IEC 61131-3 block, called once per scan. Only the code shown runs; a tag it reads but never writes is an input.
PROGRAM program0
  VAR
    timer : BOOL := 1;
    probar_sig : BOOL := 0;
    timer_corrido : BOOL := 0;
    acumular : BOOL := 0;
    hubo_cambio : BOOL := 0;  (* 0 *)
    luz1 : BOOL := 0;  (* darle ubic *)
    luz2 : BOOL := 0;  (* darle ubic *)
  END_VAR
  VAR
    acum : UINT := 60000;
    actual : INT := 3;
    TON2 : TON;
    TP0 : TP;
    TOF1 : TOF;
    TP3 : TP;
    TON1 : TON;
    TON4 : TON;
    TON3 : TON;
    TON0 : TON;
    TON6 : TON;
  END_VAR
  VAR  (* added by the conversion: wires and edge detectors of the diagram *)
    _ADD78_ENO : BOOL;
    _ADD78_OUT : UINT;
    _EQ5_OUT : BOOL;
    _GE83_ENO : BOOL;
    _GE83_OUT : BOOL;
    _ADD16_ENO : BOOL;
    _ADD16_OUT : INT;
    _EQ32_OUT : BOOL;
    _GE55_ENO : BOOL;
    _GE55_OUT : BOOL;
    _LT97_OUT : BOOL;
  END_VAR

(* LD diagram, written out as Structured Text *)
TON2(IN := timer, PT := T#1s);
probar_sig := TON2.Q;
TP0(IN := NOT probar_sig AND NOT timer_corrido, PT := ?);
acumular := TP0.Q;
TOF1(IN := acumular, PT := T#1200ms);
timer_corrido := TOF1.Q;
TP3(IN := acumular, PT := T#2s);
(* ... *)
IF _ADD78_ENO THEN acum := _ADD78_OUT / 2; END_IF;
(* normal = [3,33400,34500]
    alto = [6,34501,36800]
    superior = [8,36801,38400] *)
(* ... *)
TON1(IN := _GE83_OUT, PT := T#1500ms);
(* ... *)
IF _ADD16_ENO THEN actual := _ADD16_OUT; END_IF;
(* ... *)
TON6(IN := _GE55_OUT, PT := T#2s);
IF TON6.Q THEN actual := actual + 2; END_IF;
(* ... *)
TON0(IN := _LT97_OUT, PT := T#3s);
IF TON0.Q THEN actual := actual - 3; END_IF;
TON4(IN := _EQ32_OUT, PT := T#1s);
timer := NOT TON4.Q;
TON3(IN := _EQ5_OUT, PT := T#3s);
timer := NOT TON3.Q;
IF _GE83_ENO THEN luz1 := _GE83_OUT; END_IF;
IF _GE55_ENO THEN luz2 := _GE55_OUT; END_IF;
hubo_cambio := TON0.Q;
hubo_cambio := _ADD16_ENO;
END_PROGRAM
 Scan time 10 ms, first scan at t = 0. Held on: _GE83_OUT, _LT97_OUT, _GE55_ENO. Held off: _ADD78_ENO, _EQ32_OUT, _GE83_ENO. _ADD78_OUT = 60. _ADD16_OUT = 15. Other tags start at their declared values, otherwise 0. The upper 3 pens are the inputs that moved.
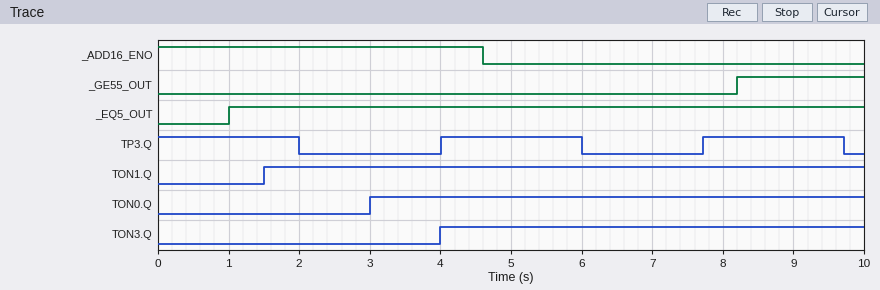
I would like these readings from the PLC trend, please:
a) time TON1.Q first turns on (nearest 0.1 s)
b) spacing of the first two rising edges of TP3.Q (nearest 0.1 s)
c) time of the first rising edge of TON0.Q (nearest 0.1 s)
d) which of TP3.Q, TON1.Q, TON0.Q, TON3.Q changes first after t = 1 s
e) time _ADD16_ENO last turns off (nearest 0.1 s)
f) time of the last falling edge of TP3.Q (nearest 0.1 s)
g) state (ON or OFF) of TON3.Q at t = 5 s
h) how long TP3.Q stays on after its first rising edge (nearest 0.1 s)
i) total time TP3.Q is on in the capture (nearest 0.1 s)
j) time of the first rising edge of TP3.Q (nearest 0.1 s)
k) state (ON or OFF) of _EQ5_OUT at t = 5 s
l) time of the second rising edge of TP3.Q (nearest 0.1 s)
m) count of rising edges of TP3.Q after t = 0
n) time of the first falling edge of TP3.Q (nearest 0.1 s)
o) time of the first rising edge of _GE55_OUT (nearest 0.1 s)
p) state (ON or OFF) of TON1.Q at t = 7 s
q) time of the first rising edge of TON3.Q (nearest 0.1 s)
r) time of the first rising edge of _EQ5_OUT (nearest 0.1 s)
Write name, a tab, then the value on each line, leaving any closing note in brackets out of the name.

time TON1.Q first turns on	1.5 s
spacing of the first two rising edges of TP3.Q	3.7 s
time of the first rising edge of TON0.Q	3.0 s
which of TP3.Q, TON1.Q, TON0.Q, TON3.Q changes first after t = 1 s	TON1.Q
time _ADD16_ENO last turns off	4.6 s
time of the last falling edge of TP3.Q	9.7 s
state (ON or OFF) of TON3.Q at t = 5 s	ON
how long TP3.Q stays on after its first rising edge	2.0 s
total time TP3.Q is on in the capture	6.0 s
time of the first rising edge of TP3.Q	4.0 s
state (ON or OFF) of _EQ5_OUT at t = 5 s	ON
time of the second rising edge of TP3.Q	7.7 s
count of rising edges of TP3.Q after t = 0	2
time of the first falling edge of TP3.Q	2.0 s
time of the first rising edge of _GE55_OUT	8.2 s
state (ON or OFF) of TON1.Q at t = 7 s	ON
time of the first rising edge of TON3.Q	4.0 s
time of the first rising edge of _EQ5_OUT	1.0 s
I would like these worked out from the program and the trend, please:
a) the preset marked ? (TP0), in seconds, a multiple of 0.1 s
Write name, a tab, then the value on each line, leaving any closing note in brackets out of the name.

the preset marked ? (TP0), in seconds, a multiple of 0.1 s	2.5 s
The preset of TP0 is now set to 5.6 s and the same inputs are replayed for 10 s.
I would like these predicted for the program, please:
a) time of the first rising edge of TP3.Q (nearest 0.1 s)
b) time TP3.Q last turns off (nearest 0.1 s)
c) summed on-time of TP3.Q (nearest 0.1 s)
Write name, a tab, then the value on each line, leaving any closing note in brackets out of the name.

time of the first rising edge of TP3.Q	6.8 s
time TP3.Q last turns off	8.8 s
summed on-time of TP3.Q	4.0 s
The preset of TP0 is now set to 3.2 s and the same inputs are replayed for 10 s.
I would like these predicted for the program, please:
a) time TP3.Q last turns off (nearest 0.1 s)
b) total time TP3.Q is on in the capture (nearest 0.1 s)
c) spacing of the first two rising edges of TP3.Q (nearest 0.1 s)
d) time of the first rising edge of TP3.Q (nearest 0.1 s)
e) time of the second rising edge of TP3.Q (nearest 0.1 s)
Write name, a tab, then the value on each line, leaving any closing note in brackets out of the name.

time TP3.Q last turns off	6.4 s
total time TP3.Q is on in the capture	5.2 s
spacing of the first two rising edges of TP3.Q	4.4 s
time of the first rising edge of TP3.Q	4.4 s
time of the second rising edge of TP3.Q	8.8 s
